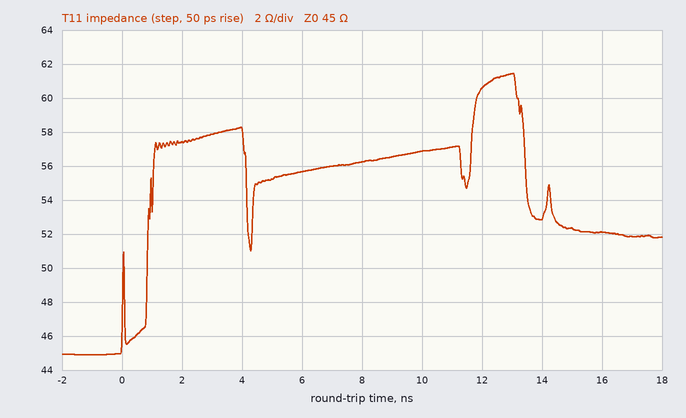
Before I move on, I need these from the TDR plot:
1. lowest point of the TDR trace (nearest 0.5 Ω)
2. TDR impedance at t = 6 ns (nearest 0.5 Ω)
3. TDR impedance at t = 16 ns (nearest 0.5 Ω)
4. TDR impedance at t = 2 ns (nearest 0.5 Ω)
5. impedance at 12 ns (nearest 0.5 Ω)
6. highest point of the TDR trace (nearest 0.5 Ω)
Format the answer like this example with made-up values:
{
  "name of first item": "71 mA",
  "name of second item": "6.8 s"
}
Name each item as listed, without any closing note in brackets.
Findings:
{
  "lowest point of the TDR trace": "45.0 Ω",
  "TDR impedance at t = 6 ns": "55.5 Ω",
  "TDR impedance at t = 16 ns": "52.0 Ω",
  "TDR impedance at t = 2 ns": "57.5 Ω",
  "impedance at 12 ns": "60.5 Ω",
  "highest point of the TDR trace": "61.5 Ω"
}
